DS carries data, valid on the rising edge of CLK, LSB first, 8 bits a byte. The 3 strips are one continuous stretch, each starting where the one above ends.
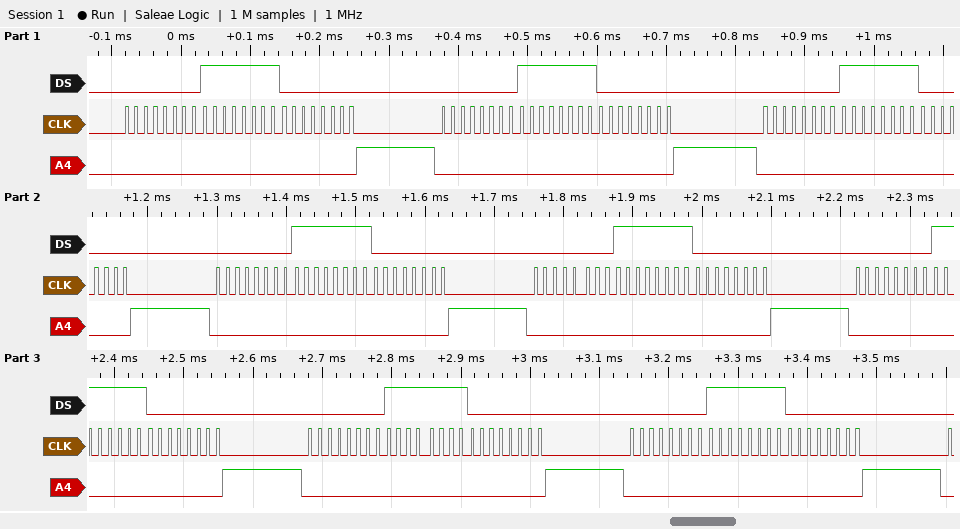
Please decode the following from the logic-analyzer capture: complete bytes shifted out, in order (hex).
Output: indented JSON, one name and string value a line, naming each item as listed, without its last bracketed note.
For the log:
{
  "complete bytes shifted out, in order": "00 FF 00 00 FF 00 00 FF 00 00 FF 00 00 FF 00 00 FF 00 00 FF 00 00 FF 00"
}
